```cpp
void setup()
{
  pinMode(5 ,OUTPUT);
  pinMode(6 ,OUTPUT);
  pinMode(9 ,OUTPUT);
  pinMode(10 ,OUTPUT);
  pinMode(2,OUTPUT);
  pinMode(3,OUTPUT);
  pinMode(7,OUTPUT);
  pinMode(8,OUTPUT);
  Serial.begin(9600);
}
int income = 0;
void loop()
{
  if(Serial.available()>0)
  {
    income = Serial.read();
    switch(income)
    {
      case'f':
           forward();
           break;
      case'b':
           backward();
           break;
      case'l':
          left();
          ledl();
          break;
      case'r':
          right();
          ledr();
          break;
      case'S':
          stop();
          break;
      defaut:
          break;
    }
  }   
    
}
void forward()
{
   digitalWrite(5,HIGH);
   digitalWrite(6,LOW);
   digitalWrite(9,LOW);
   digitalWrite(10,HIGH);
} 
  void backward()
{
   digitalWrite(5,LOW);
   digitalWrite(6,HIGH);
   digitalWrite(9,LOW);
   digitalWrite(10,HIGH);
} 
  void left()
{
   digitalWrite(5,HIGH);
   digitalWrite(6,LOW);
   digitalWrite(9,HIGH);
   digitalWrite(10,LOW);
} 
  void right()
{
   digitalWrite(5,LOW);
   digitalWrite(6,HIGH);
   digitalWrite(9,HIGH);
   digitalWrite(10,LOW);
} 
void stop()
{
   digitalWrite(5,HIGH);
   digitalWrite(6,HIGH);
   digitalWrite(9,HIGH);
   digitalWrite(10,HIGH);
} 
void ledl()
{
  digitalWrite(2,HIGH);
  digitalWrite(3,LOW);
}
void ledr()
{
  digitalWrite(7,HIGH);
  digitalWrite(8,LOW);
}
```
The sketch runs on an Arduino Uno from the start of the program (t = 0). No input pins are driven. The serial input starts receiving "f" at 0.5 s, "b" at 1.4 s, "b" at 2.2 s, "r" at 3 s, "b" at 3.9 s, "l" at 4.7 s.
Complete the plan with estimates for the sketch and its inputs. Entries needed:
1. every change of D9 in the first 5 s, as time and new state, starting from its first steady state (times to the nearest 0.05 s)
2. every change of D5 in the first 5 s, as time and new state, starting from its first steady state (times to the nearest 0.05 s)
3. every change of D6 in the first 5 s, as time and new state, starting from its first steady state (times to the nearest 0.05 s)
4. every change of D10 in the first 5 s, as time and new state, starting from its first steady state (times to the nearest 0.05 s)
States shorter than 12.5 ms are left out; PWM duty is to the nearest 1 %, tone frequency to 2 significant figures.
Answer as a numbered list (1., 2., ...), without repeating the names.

1. 0 s low; 3 s high; 3.9 s low; 4.7 s high
2. 0 s low; 0.5 s high; 1.4 s low; 4.7 s high
3. 0 s low; 1.4 s high; 4.7 s low
4. 0 s low; 0.5 s high; 3 s low; 3.9 s high; 4.7 s low
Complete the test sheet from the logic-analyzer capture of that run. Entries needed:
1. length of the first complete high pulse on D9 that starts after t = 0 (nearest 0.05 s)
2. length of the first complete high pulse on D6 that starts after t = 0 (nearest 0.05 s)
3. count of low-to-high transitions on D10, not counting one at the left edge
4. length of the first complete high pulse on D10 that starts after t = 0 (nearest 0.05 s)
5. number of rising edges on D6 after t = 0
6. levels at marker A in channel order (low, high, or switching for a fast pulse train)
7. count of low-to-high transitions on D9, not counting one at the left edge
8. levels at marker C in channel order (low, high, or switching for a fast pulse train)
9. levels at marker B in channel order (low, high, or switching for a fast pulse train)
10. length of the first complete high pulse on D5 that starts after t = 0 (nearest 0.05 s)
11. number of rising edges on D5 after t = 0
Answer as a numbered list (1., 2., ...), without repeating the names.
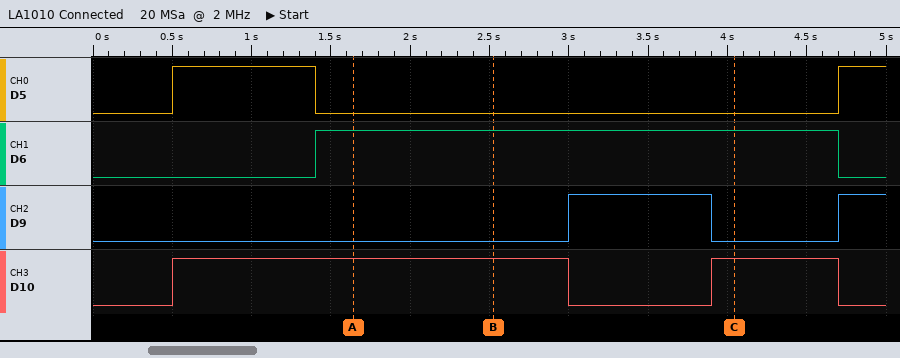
1. 0.90 s
2. 3.30 s
3. 2
4. 2.50 s
5. 1
6. D5 low, D6 high, D9 low, D10 high
7. 2
8. D5 low, D6 high, D9 low, D10 high
9. D5 low, D6 high, D9 low, D10 high
10. 0.90 s
11. 2
